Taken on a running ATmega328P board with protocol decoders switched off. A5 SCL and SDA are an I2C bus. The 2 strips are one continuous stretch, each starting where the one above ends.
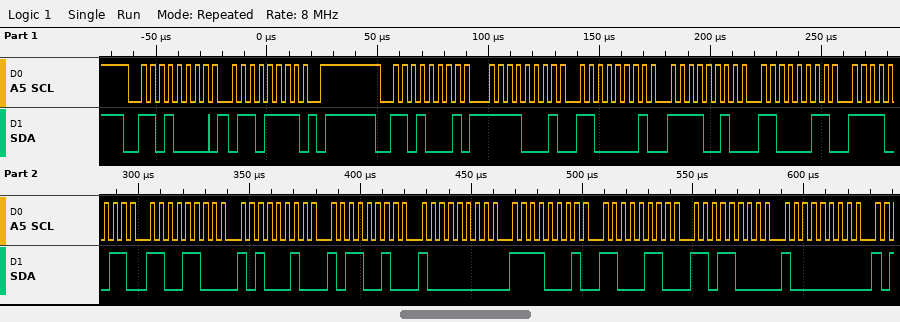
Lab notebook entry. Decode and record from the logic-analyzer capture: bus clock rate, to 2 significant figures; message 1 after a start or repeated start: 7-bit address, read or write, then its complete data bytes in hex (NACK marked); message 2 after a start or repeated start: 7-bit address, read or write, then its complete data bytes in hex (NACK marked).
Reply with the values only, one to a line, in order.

250 kHz
0x68 write: 6F
0x68 read: F1 C1 F2 C3 F3 CC A2 B2 80 F1 C6 D8 80
